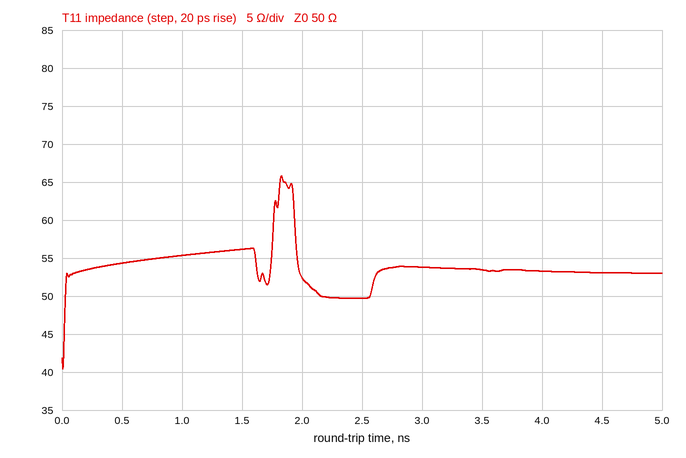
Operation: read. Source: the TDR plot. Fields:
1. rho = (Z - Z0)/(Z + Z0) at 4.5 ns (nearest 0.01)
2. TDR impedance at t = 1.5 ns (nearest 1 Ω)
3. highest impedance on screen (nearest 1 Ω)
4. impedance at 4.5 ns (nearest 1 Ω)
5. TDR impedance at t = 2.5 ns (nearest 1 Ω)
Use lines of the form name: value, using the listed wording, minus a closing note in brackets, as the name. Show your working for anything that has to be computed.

rho = (Z - Z0)/(Z + Z0) at 4.5 ns: (53 − 50)/(53 + 50) ≈ +0.03
TDR impedance at t = 1.5 ns: 56 Ω
highest impedance on screen: 66 Ω
impedance at 4.5 ns: 53 Ω
TDR impedance at t = 2.5 ns: 50 Ω
